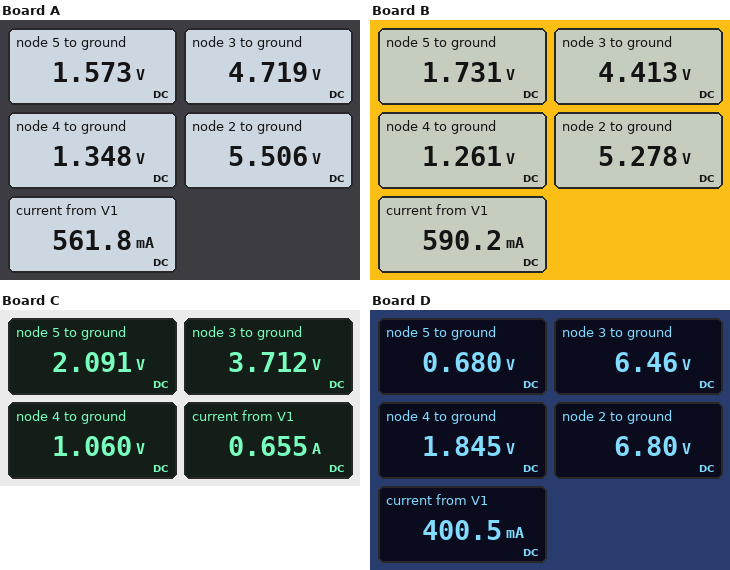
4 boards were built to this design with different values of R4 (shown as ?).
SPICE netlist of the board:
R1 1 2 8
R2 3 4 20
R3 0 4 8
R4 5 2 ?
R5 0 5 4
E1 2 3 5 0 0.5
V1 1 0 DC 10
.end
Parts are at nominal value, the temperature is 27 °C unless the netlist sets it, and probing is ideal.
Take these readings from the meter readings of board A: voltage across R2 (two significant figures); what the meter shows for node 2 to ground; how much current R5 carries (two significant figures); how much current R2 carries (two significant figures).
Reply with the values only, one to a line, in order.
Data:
3.4 V
5.506 V
390 mA
170 mA
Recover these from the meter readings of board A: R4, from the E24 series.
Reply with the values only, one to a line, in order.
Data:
10 Ω
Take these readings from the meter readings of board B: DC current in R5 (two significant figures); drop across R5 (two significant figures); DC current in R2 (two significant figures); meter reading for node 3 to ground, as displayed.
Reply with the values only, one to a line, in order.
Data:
430 mA
1.7 V
160 mA
4.413 V
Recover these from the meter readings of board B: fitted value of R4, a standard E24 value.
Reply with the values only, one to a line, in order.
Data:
8.2 Ω
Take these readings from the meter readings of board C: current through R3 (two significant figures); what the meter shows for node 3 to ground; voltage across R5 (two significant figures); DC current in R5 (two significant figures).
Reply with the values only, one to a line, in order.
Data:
130 mA
3.712 V
2.1 V
520 mA
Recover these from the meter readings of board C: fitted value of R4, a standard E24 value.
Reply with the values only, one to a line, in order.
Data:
5.1 Ω
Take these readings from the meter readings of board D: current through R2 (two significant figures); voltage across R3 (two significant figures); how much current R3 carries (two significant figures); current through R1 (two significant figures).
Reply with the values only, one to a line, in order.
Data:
230 mA
1.8 V
230 mA
400 mA
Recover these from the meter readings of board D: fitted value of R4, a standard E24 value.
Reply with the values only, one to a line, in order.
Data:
36 Ω
